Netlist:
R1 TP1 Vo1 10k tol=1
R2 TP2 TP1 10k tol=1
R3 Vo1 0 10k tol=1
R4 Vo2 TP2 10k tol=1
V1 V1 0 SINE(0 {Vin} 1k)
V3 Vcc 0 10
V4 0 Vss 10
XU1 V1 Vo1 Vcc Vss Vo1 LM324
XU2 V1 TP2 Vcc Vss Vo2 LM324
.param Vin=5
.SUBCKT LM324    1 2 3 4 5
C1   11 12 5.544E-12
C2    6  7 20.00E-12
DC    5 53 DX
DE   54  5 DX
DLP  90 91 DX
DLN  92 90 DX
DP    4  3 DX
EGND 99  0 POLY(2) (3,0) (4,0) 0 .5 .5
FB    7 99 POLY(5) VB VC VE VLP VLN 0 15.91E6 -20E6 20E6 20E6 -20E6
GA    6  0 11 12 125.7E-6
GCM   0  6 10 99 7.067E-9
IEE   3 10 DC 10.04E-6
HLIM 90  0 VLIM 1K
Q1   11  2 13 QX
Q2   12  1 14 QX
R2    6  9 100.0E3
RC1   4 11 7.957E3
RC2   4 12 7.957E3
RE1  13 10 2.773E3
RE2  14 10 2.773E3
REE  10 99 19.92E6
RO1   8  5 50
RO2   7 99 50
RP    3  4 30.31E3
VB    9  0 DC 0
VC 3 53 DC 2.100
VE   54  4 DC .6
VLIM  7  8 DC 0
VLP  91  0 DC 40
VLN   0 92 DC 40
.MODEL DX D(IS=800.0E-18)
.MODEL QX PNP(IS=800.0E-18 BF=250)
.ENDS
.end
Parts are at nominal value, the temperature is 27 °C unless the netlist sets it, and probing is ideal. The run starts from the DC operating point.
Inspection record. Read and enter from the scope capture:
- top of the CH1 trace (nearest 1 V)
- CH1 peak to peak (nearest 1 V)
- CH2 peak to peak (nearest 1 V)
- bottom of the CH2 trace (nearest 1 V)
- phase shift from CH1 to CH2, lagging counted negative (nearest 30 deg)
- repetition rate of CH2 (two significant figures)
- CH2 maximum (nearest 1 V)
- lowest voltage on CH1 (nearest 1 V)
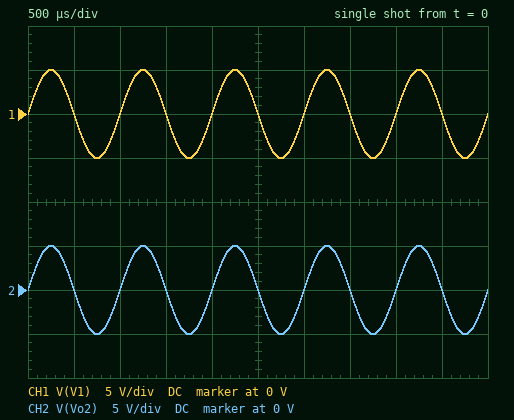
5 V
10 V
10 V
-5 V
0 deg
1.0 kHz
5 V
-5 V
